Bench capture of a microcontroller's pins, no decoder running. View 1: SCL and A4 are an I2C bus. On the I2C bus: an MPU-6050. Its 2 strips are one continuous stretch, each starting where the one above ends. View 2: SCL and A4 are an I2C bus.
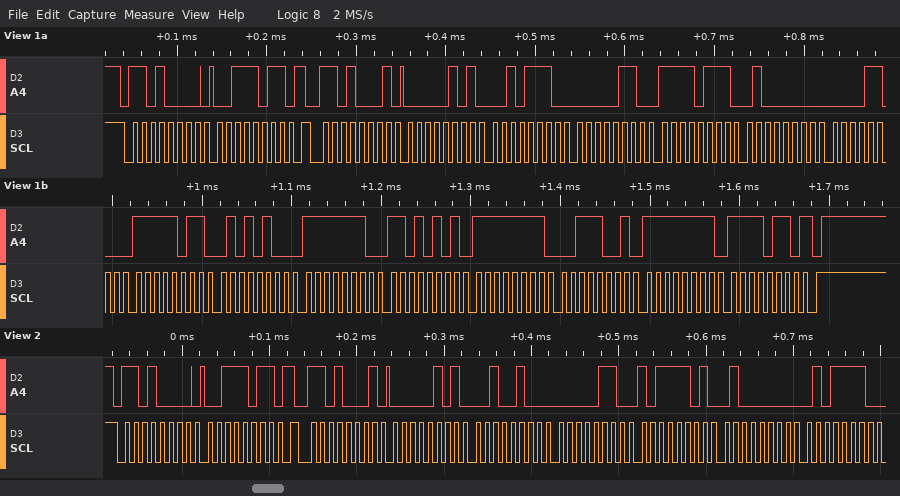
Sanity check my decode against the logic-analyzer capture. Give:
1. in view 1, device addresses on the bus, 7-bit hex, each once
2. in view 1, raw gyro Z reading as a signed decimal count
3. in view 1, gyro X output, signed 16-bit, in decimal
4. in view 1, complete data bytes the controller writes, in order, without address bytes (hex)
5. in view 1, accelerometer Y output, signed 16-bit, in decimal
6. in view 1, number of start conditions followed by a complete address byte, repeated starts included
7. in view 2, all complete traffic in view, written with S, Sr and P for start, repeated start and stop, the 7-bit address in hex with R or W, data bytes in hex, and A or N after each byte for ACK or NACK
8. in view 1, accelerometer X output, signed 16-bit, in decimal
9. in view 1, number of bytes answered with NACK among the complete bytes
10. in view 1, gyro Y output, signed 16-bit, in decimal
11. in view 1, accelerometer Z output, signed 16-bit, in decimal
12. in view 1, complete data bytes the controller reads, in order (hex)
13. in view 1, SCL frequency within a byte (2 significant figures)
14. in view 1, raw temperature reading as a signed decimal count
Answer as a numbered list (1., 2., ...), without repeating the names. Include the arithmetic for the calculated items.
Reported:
1. 0x68
2. 0xFFF6 = -10
3. 0xFED5 = -299
4. 3B
5. 0x06F7 = 1783
6. 2
7. S 68W A 3B A Sr 68R A 05 A 24 A 06 A BD A 40 A 5E A
8. 0x052E = 1326
9. 1
10. 0xFF39 = -199
11. 0x400C = 16396
12. 05 2E 06 F7 40 0C FB 54 FE D5 FF 39 FF F6
13. 100 kHz
14. 0xFB54 = -1196
